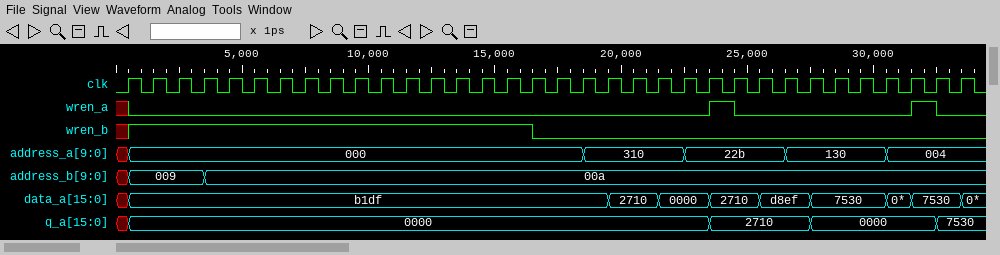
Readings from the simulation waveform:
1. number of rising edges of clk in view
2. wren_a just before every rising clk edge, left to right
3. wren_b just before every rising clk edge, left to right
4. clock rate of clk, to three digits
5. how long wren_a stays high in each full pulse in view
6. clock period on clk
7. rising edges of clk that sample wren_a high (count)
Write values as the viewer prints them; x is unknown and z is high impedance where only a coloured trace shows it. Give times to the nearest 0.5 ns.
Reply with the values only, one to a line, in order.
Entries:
34
x 0 0 0 0 0 0 0 0 0 0 0 0 0 0 0 0 0 0 0 0 0 0 0 1 0 0 0 0 0 0 0 1 0
x 1 1 1 1 1 1 1 1 1 1 1 1 1 1 1 1 0 0 0 0 0 0 0 0 0 0 0 0 0 0 0 0 0
1.00 GHz
1 ns, 1 ns
1 ns
2
